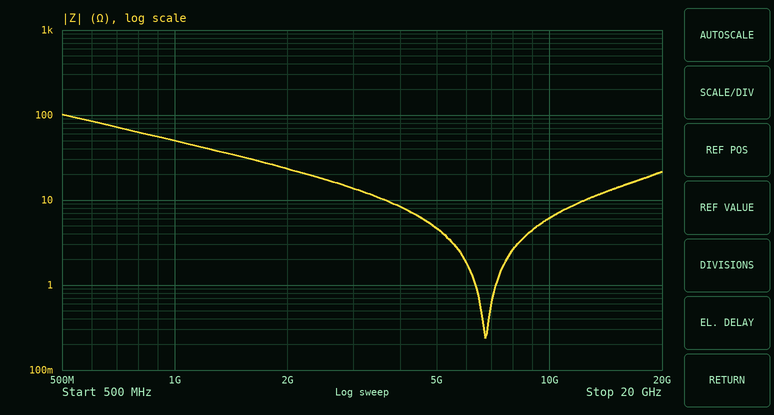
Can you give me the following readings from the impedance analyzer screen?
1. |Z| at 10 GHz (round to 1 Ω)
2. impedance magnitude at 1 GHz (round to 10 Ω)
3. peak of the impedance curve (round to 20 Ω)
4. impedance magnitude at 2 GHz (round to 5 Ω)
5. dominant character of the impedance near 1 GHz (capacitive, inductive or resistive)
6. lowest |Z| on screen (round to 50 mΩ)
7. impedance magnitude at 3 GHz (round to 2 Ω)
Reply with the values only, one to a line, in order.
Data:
6 Ω
50 Ω
100 Ω
25 Ω
capacitive
250 mΩ
14 Ω
